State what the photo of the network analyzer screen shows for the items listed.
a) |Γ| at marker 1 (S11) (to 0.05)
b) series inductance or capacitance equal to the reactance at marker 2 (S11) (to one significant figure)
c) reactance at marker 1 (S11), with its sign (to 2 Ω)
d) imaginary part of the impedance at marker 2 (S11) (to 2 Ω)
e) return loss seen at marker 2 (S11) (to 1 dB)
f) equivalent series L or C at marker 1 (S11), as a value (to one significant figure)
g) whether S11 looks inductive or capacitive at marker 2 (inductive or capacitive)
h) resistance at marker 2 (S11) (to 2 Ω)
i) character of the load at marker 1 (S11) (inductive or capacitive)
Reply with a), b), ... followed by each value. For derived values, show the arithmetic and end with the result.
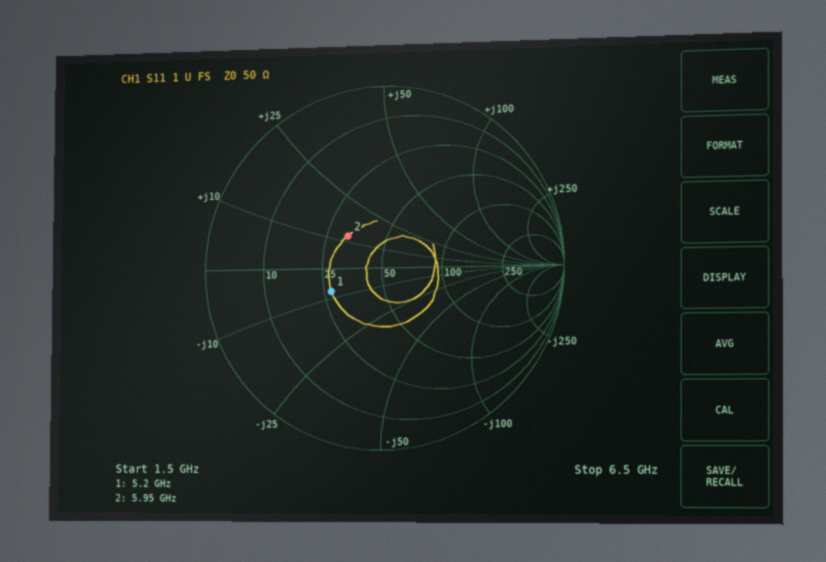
a) 0.30
b) L = 12 Ω/(2π × 5.95 GHz) ≈ 321 pH, so 300 pH to one significant figure
c) -8 Ω
d) +12 Ω
e) 12 dB
f) C = 1/(2π × 5.2 GHz × 8 Ω) ≈ 4 pF
g) inductive
h) 32 Ω
i) capacitive
